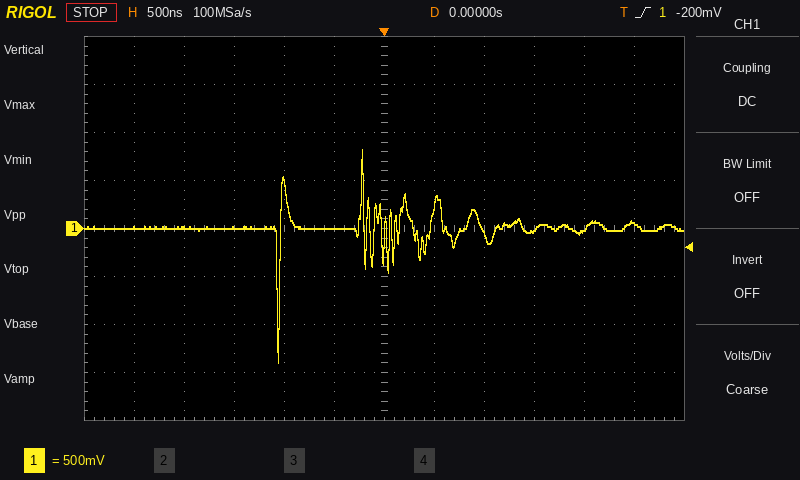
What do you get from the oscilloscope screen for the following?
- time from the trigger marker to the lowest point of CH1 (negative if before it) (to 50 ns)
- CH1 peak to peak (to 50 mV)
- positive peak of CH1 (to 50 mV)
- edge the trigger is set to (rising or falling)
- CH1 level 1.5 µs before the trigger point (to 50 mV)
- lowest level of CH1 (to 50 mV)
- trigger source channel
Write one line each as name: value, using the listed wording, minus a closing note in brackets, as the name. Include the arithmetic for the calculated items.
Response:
time from the trigger marker to the lowest point of CH1 (negative if before it): -1.05 µs
CH1 peak to peak: 800 mV − (-1.40 V) = 2.20 V
positive peak of CH1: 800 mV
edge the trigger is set to: rising
CH1 level 1.5 µs before the trigger point: 0 mV
lowest level of CH1: -1.40 V
trigger source channel: CH1
